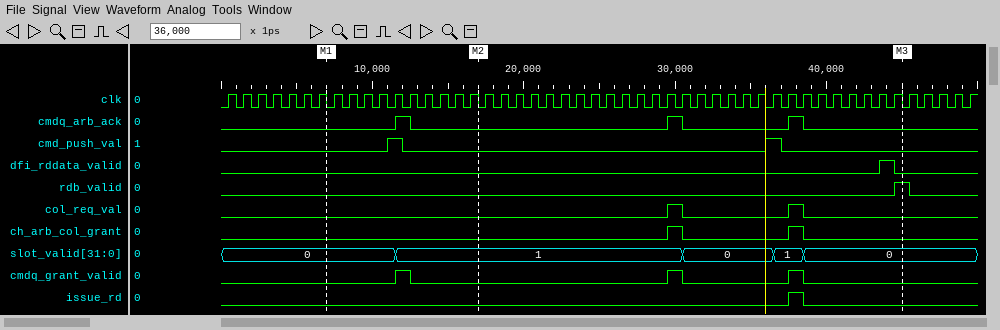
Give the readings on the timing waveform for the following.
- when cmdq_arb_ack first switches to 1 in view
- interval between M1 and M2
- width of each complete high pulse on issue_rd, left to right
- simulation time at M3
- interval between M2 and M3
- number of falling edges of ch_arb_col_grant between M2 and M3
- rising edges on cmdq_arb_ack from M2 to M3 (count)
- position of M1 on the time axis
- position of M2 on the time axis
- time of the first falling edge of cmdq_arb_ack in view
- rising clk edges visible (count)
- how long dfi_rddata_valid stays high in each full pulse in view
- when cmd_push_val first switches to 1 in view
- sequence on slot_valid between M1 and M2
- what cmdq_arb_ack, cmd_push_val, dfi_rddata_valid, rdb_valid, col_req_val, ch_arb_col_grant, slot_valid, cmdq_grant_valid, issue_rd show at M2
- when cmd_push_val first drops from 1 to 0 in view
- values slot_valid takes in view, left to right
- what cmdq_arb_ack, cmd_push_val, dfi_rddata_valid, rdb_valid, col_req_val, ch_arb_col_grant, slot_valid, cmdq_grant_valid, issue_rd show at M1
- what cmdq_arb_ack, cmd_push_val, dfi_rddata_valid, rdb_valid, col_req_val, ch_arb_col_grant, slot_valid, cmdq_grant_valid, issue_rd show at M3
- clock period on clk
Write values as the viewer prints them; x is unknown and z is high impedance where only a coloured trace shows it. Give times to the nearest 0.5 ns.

11.5 ns
10 ns
1 ns
45 ns
28 ns
2
2
7 ns
17 ns
12.5 ns
50
1 ns
11 ns
0, 1
cmdq_arb_ack=0, cmd_push_val=0, dfi_rddata_valid=0, rdb_valid=0, col_req_val=0, ch_arb_col_grant=0, slot_valid=1, cmdq_grant_valid=0, issue_rd=0
12 ns
0, 1, 0, 1, 0
cmdq_arb_ack=0, cmd_push_val=0, dfi_rddata_valid=0, rdb_valid=0, col_req_val=0, ch_arb_col_grant=0, slot_valid=0, cmdq_grant_valid=0, issue_rd=0
cmdq_arb_ack=0, cmd_push_val=0, dfi_rddata_valid=0, rdb_valid=1, col_req_val=0, ch_arb_col_grant=0, slot_valid=0, cmdq_grant_valid=0, issue_rd=0
1 ns
